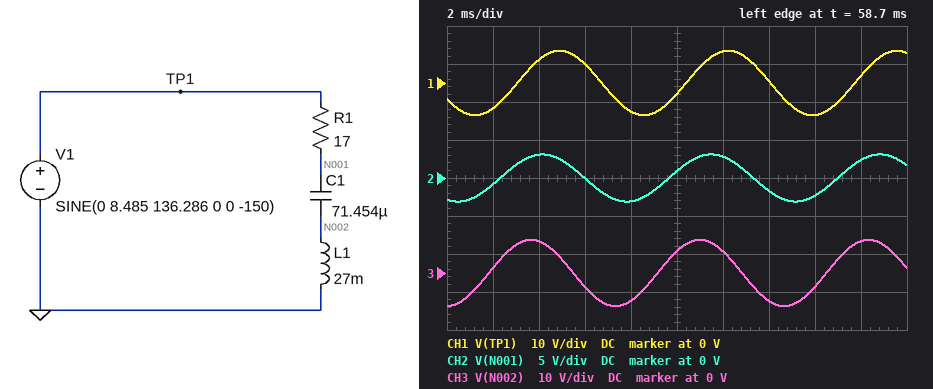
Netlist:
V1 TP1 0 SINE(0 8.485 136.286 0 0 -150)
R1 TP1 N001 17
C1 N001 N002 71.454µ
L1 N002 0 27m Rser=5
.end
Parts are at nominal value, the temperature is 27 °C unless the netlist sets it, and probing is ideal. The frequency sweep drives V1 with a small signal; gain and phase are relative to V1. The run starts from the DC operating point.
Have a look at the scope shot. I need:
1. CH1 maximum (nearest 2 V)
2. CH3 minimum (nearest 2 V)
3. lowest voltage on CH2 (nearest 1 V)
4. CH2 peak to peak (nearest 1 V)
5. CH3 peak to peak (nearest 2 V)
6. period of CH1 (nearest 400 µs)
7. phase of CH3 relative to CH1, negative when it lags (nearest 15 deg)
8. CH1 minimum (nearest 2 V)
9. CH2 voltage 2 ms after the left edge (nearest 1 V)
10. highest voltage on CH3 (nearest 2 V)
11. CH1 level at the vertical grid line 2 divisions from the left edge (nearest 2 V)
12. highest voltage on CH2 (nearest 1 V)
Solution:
8 V
-8 V
-3 V
6 V
18 V
7.2 ms
60 deg
-8 V
-1 V
8 V
6 V
3 V
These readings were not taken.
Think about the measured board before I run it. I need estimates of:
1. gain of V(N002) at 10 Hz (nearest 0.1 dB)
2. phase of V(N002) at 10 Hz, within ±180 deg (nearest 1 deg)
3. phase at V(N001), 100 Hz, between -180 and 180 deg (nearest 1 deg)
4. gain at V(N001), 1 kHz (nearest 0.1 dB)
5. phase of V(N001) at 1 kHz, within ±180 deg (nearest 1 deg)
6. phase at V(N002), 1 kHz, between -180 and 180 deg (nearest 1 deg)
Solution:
-32.5 dB
103 deg
-33 deg
-0.1 dB
6 deg
6 deg
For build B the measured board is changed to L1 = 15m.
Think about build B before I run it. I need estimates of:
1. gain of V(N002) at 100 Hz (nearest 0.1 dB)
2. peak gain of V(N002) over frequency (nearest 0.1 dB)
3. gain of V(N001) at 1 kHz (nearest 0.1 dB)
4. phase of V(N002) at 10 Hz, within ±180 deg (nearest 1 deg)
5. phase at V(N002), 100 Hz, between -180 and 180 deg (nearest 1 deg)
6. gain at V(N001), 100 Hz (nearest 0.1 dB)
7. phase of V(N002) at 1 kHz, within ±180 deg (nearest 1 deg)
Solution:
-7.6 dB
0 dB
-0.2 dB
95 deg
92 deg
-5.3 dB
10 deg
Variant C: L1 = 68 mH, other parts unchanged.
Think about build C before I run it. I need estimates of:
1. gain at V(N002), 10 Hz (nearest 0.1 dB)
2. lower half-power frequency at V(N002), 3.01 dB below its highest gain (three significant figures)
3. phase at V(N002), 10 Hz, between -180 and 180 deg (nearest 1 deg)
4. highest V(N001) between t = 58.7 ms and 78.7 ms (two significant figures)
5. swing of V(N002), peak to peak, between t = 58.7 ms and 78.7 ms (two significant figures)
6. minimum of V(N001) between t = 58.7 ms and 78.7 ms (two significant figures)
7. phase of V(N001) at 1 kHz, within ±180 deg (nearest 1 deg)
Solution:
-30.5 dB
60.5 Hz
125 deg
7.6 V
21 V
-7.6 V
2 deg
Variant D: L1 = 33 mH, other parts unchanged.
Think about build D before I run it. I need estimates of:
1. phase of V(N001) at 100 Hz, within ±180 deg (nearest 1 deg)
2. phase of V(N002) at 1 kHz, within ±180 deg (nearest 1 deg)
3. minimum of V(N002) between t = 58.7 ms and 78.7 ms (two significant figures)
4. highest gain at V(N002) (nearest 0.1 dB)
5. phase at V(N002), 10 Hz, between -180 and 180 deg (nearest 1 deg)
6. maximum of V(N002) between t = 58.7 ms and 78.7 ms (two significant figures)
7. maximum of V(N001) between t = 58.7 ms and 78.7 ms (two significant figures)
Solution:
-13 deg
5 deg
-9.7 V
1.2 dB
107 deg
9.7 V
4.4 V
